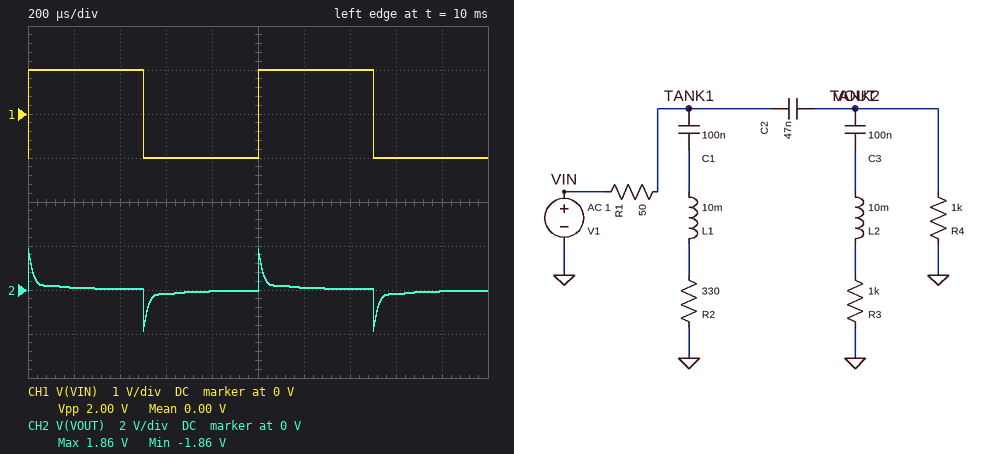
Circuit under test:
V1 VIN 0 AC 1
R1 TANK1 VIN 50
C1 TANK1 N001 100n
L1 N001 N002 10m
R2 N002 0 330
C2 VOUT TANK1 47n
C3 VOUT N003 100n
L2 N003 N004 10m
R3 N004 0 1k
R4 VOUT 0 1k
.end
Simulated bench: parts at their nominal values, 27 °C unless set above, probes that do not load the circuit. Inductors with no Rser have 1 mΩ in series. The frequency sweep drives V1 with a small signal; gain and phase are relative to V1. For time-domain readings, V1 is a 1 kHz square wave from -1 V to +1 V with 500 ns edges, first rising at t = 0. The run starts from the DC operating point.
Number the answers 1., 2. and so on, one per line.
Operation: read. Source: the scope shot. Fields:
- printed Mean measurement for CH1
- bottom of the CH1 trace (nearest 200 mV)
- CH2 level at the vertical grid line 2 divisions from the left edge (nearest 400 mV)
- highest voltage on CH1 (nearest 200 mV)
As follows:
1. 0.00 V
2. -1.0 V
3. 0 V
4. 1.0 V
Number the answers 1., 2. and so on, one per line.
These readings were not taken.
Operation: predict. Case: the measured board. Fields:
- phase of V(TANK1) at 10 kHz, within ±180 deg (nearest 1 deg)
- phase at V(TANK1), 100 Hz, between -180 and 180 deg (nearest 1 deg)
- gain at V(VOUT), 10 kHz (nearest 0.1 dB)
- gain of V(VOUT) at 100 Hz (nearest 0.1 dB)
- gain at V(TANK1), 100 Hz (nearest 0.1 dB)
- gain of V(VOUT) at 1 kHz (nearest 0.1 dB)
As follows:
1. 2 deg
2. 0 deg
3. -1.6 dB
4. -30.7 dB
5. 0 dB
6. -14.2 dB
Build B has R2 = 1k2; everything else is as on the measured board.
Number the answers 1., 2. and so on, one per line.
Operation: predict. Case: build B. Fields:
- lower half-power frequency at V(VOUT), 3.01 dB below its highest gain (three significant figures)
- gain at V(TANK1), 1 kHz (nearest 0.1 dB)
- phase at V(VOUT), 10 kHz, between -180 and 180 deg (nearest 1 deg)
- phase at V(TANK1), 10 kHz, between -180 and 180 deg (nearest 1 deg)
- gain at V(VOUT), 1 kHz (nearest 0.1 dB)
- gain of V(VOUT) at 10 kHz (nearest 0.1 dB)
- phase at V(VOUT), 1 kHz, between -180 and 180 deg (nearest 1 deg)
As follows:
1. 6.76 kHz
2. -0.2 dB
3. 34 deg
4. -1 deg
5. -14.3 dB
6. -1.5 dB
7. 58 deg
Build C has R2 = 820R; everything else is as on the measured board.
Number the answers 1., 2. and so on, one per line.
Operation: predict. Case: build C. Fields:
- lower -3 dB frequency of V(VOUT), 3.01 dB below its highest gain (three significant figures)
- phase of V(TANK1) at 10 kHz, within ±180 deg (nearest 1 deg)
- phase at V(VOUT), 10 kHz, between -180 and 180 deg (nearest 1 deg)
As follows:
1. 6.94 kHz
2. 0 deg
3. 35 deg
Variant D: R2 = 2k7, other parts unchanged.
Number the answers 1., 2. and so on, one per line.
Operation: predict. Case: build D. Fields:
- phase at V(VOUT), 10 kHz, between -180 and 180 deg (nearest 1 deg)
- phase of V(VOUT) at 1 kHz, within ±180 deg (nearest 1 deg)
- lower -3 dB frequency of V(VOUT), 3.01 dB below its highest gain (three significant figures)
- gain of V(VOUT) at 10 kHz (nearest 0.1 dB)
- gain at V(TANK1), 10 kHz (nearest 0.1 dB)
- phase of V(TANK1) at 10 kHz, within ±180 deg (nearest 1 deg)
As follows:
1. 34 deg
2. 59 deg
3. 6.58 kHz
4. -1.4 dB
5. -0.8 dB
6. -2 deg
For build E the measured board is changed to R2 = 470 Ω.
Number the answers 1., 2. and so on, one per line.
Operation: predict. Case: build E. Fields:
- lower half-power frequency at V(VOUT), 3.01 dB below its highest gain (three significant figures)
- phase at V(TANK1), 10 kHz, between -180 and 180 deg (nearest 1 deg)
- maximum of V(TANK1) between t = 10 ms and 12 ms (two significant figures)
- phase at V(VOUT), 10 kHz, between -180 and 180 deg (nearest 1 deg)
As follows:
1. 7.26 kHz
2. 1 deg
3. 1.0 V
4. 36 deg
